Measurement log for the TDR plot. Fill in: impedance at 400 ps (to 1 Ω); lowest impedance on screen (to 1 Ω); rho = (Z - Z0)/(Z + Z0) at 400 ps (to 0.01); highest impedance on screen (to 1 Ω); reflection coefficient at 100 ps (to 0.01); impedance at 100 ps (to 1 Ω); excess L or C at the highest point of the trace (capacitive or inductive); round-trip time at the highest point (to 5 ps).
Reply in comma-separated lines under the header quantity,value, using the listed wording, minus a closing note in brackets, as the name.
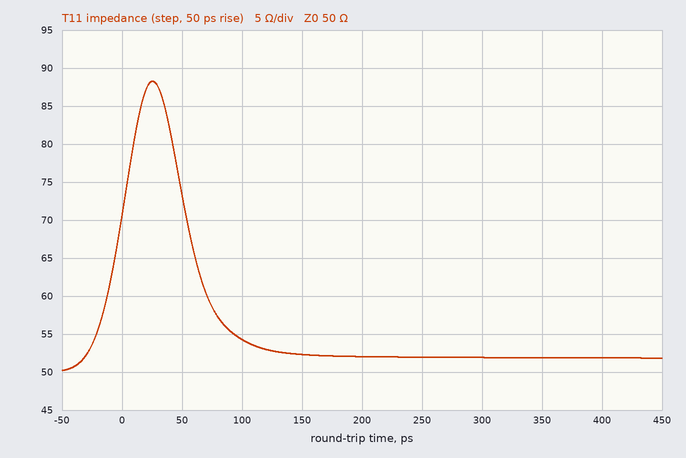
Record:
quantity,value
impedance at 400 ps,52 Ω
lowest impedance on screen,50 Ω
rho = (Z - Z0)/(Z + Z0) at 400 ps,+0.02
highest impedance on screen,88 Ω
reflection coefficient at 100 ps,+0.04
impedance at 100 ps,54 Ω
excess L or C at the highest point of the trace,inductive
round-trip time at the highest point,25 ps
